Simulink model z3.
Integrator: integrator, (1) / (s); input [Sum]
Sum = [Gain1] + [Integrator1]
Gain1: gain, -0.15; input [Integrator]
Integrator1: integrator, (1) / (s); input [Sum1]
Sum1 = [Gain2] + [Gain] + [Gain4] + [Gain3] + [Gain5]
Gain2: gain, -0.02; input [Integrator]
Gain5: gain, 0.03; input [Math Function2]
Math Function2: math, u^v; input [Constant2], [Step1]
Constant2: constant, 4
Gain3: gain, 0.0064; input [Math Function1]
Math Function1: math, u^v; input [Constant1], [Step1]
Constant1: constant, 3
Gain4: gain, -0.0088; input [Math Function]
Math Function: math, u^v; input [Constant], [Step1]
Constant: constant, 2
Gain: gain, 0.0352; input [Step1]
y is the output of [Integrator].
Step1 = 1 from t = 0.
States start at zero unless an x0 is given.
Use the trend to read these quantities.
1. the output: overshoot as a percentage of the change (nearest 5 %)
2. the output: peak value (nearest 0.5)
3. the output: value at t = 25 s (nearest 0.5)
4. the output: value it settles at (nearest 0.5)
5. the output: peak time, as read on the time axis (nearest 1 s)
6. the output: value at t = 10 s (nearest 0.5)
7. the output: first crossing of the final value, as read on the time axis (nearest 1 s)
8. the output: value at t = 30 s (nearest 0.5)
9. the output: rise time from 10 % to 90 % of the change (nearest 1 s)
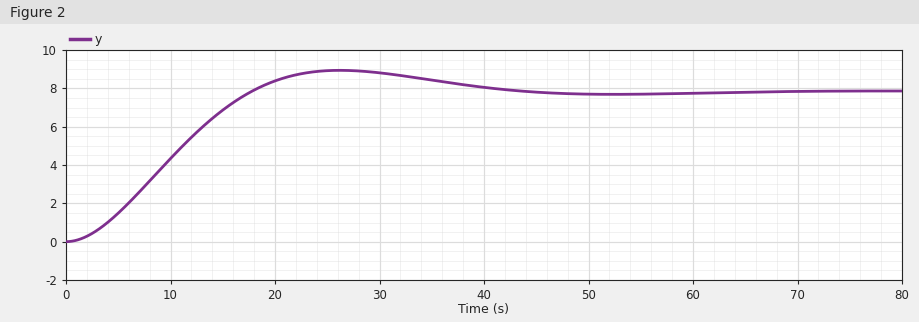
15 %
9.0
9.0
8.0
26 s
4.5
18 s
9.0
12 s
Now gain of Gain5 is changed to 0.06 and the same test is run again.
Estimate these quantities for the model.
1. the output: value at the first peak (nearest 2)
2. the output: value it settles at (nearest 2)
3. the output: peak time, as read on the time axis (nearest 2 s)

16
14
26 s
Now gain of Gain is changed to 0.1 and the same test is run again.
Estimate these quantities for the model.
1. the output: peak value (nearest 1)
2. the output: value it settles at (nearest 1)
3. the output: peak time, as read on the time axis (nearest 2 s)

13
11
26 s
